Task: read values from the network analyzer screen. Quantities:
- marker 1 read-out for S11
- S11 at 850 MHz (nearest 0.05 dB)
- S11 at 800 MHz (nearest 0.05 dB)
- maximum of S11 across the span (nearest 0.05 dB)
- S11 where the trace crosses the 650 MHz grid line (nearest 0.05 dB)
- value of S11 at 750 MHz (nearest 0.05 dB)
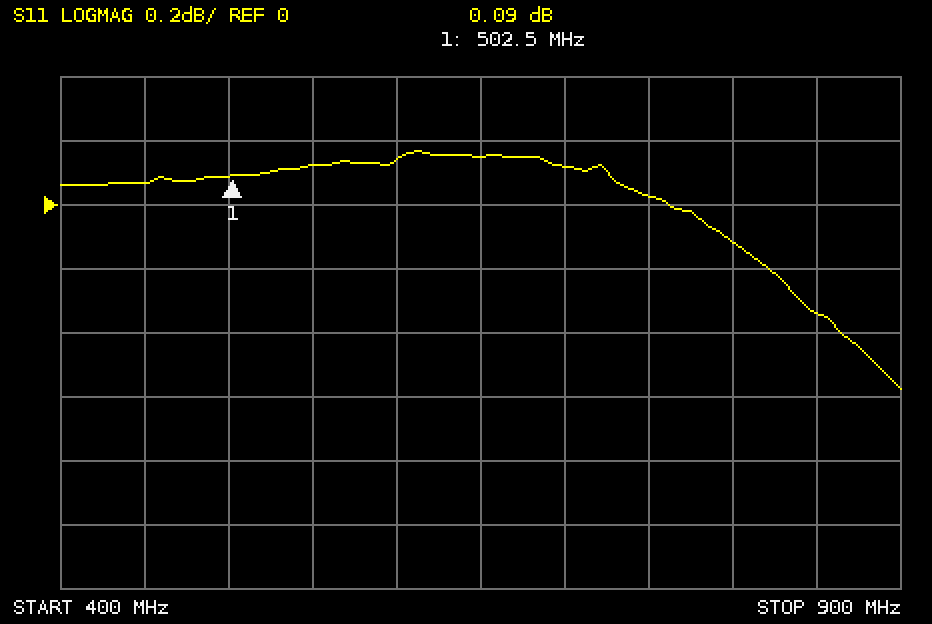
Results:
0.09 dB
-0.35 dB
-0.10 dB
0.15 dB
0.15 dB
0.05 dB
